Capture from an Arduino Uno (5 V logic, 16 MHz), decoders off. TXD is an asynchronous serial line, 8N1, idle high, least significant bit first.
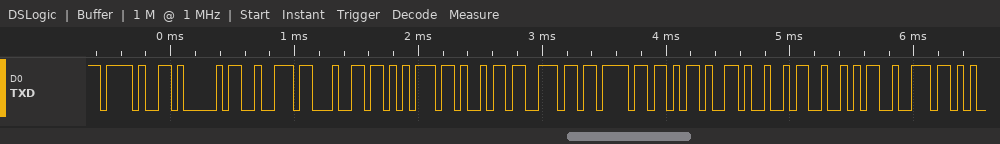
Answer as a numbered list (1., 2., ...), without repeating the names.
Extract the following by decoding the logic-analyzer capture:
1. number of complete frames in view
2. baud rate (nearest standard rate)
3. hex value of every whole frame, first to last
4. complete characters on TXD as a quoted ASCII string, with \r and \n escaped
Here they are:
1. 12
2. 19200 baud
3. 2F 41 72 64 75 69 6E 6F 2D 49 52 72
4. "/Arduino-IRr"
